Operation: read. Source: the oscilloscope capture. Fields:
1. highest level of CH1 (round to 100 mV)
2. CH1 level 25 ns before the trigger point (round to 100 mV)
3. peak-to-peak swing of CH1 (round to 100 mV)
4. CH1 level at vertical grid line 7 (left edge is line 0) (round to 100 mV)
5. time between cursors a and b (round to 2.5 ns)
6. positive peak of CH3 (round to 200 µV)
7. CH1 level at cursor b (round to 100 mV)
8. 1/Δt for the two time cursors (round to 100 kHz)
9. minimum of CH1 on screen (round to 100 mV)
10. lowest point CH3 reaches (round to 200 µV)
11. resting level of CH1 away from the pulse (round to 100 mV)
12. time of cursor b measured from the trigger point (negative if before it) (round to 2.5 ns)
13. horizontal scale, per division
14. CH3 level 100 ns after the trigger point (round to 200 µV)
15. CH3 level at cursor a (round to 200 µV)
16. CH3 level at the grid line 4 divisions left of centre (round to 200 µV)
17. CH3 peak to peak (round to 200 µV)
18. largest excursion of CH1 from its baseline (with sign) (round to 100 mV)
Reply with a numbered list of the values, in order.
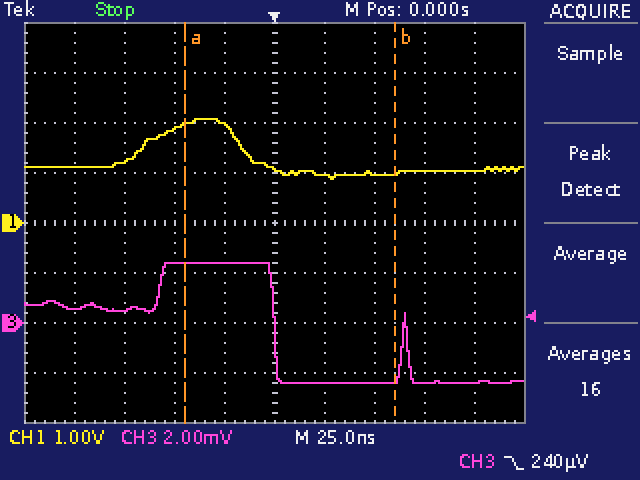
1. 2.1 V
2. 2.0 V
3. 1.2 V
4. 1.0 V
5. 105.0 ns
6. 2.4 mV
7. 1.0 V
8. 9.5 MHz
9. 900 mV
10. -2.4 mV
11. 1.1 V
12. +60.0 ns
13. 25 ns
14. -2.4 mV
15. 2.4 mV
16. 600 µV
17. 4.8 mV
18. +1.0 V
